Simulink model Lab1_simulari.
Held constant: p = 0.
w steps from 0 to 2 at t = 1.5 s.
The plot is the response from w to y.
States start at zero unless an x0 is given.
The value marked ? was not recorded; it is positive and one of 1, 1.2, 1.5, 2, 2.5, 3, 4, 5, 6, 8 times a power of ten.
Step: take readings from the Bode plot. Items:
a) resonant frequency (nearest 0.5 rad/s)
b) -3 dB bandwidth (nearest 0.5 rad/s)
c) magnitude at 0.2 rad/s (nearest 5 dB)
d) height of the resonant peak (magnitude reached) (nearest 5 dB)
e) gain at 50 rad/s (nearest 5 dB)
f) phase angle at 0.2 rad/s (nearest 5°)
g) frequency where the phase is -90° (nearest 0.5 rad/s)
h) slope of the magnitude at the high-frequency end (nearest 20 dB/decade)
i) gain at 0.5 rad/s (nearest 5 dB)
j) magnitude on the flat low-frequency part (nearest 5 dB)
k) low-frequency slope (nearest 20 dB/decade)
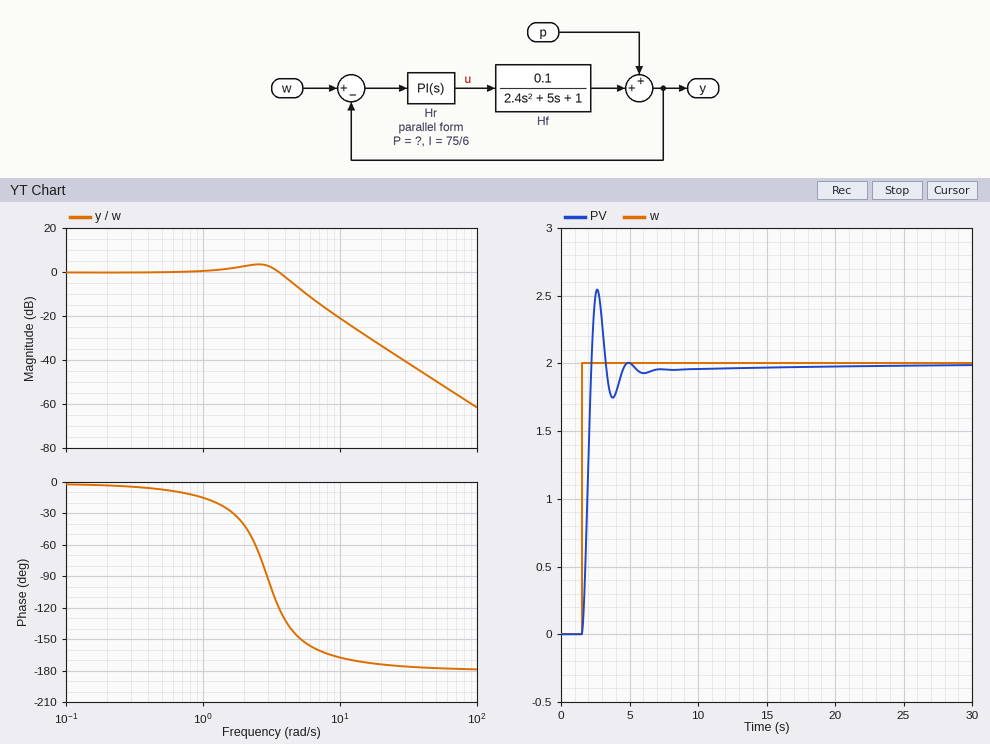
2.5 rad/s
4.0 rad/s
0 dB
5 dB
-50 dB
-5°
3.0 rad/s
-40 dB/decade
0 dB
0 dB
0 dB/decade
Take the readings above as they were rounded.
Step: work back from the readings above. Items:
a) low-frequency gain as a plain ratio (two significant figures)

1.0
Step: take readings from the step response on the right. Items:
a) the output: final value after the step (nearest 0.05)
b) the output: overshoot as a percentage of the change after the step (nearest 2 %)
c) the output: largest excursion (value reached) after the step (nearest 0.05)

2.00
28 %
2.55
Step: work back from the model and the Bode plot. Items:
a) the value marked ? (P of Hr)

200
